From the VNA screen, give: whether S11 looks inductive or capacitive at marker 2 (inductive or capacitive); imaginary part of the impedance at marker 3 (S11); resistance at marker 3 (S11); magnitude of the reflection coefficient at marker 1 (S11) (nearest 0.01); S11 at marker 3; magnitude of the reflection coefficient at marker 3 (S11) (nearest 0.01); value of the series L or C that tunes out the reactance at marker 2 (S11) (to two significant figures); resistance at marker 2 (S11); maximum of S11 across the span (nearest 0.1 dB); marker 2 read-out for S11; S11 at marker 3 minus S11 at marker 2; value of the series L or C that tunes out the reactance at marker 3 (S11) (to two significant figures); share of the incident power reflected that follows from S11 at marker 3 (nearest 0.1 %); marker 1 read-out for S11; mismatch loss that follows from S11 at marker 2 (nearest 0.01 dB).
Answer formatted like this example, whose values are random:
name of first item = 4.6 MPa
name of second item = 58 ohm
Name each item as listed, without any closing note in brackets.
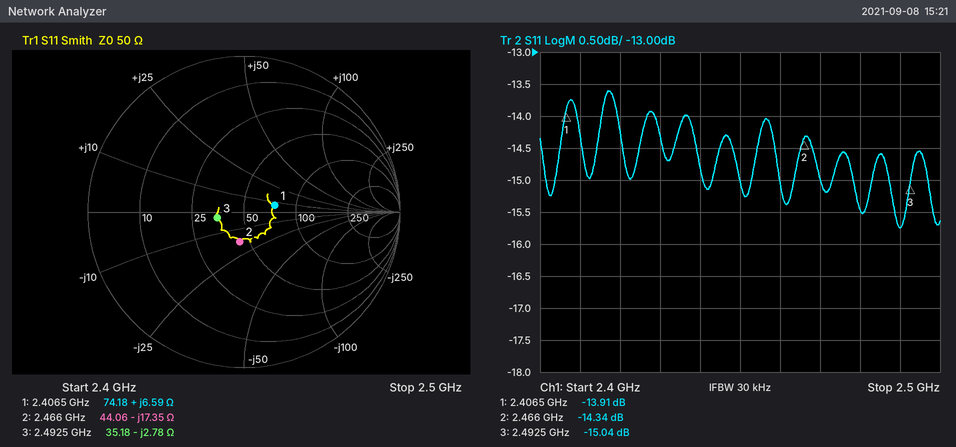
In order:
whether S11 looks inductive or capacitive at marker 2 = capacitive
imaginary part of the impedance at marker 3 = -2.78 Ω
resistance at marker 3 = 35.18 Ω
magnitude of the reflection coefficient at marker 1 (S11) = 0.20
S11 at marker 3 = -15.04 dB
magnitude of the reflection coefficient at marker 3 (S11) = 0.18
value of the series L or C that tunes out the reactance at marker 2 (S11) = 1.1 nH
resistance at marker 2 = 44.06 Ω
maximum of S11 across the span = -13.6 dB
marker 2 read-out for S11 = -14.34 dB
S11 at marker 3 minus S11 at marker 2 = -0.70 dB
value of the series L or C that tunes out the reactance at marker 3 (S11) = 180 pH
share of the incident power reflected that follows from S11 at marker 3 = 3.1 %
marker 1 read-out for S11 = -13.91 dB
mismatch loss that follows from S11 at marker 2 = 0.16 dB
